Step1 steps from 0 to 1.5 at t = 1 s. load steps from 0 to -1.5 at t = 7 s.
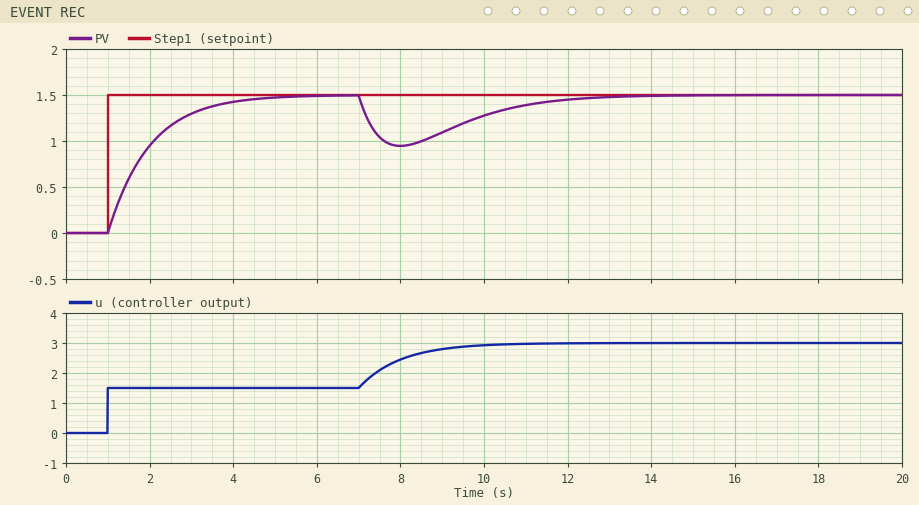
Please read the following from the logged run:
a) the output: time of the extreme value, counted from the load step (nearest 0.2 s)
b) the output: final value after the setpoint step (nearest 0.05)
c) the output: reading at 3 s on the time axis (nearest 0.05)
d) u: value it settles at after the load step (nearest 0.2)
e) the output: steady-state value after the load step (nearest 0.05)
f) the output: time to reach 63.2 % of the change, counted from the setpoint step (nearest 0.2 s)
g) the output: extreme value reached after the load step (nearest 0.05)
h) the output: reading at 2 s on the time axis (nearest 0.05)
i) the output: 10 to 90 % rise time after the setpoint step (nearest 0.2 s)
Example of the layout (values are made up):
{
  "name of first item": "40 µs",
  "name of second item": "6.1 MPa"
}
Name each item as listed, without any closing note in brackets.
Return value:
{
  "the output: time of the extreme value, counted from the load step": "1.0 s",
  "the output: final value after the setpoint step": "1.50",
  "the output: reading at 3 s on the time axis": "1.30",
  "u: value it settles at after the load step": "3.0",
  "the output: steady-state value after the load step": "1.50",
  "the output: time to reach 63.2 % of the change, counted from the setpoint step": "1.0 s",
  "the output: extreme value reached after the load step": "0.95",
  "the output: reading at 2 s on the time axis": "0.95",
  "the output: 10 to 90 % rise time after the setpoint step": "2.2 s"
}
